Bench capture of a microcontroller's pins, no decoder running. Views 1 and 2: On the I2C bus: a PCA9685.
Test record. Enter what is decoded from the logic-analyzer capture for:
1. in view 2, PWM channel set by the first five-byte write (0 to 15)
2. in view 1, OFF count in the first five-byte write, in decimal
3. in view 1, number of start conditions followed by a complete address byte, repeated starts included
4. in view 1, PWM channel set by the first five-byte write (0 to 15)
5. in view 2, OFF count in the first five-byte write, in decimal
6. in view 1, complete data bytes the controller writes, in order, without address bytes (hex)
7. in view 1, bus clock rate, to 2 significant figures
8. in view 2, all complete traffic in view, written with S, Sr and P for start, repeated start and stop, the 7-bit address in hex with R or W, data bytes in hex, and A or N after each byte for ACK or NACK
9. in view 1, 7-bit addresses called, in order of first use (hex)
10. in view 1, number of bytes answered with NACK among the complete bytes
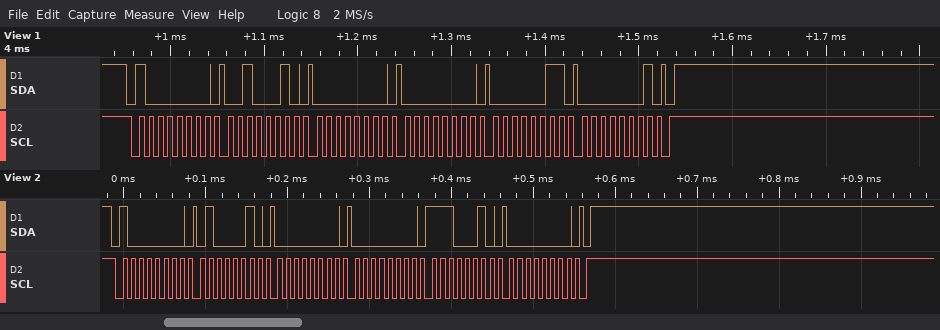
15
259
1
7
226
22 00 00 03 01
100 kHz
S 40W A 42 A 00 A 00 A E2 A 00 A P
0x40
0
